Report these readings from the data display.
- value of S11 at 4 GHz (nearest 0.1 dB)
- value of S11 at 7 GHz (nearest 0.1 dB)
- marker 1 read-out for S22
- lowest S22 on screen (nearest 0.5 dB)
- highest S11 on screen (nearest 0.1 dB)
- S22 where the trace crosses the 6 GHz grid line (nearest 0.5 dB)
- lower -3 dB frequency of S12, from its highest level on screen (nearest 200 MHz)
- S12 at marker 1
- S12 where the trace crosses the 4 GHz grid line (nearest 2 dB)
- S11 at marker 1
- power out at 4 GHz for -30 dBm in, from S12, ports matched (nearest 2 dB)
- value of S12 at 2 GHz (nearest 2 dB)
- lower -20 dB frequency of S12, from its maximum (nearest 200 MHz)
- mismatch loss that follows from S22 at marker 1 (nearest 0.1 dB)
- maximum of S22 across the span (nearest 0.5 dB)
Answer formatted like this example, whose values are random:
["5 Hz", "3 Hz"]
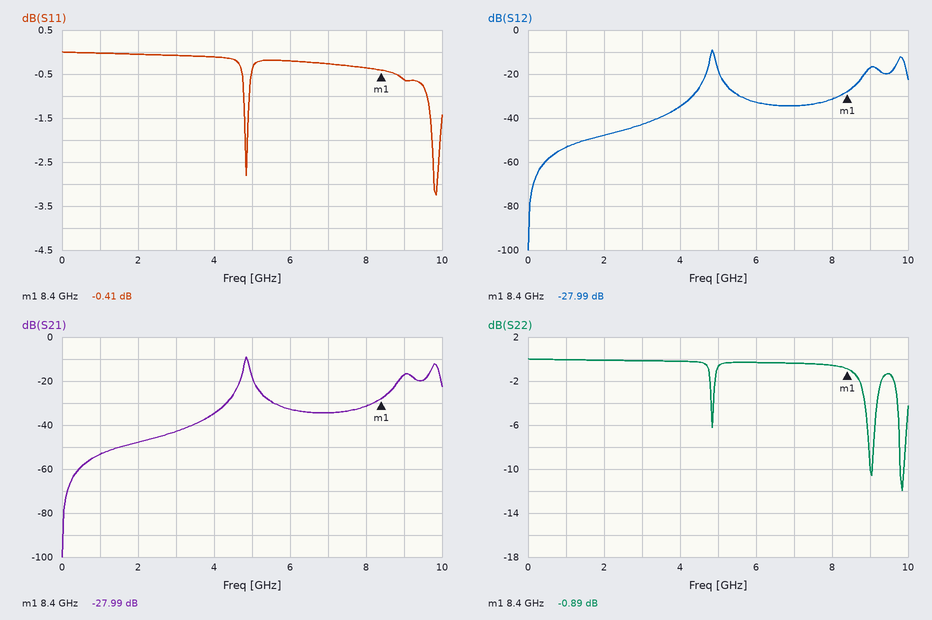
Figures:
["-0.1 dB", "-0.3 dB", "-0.89 dB", "-12.0 dB", "0.0 dB", "-0.5 dB", "4.8 GHz", "-27.99 dB", "-34 dB", "-0.41 dB", "-64 dBm", "-48 dB", "4.4 GHz", "7.3 dB", "0.0 dB"]
